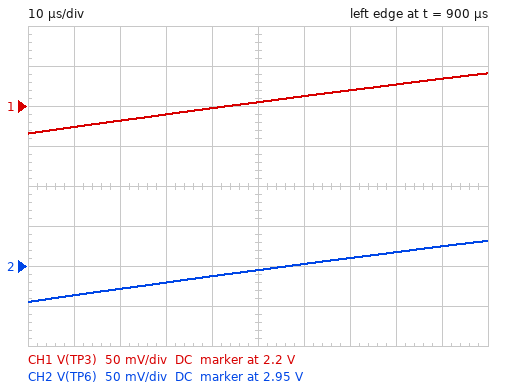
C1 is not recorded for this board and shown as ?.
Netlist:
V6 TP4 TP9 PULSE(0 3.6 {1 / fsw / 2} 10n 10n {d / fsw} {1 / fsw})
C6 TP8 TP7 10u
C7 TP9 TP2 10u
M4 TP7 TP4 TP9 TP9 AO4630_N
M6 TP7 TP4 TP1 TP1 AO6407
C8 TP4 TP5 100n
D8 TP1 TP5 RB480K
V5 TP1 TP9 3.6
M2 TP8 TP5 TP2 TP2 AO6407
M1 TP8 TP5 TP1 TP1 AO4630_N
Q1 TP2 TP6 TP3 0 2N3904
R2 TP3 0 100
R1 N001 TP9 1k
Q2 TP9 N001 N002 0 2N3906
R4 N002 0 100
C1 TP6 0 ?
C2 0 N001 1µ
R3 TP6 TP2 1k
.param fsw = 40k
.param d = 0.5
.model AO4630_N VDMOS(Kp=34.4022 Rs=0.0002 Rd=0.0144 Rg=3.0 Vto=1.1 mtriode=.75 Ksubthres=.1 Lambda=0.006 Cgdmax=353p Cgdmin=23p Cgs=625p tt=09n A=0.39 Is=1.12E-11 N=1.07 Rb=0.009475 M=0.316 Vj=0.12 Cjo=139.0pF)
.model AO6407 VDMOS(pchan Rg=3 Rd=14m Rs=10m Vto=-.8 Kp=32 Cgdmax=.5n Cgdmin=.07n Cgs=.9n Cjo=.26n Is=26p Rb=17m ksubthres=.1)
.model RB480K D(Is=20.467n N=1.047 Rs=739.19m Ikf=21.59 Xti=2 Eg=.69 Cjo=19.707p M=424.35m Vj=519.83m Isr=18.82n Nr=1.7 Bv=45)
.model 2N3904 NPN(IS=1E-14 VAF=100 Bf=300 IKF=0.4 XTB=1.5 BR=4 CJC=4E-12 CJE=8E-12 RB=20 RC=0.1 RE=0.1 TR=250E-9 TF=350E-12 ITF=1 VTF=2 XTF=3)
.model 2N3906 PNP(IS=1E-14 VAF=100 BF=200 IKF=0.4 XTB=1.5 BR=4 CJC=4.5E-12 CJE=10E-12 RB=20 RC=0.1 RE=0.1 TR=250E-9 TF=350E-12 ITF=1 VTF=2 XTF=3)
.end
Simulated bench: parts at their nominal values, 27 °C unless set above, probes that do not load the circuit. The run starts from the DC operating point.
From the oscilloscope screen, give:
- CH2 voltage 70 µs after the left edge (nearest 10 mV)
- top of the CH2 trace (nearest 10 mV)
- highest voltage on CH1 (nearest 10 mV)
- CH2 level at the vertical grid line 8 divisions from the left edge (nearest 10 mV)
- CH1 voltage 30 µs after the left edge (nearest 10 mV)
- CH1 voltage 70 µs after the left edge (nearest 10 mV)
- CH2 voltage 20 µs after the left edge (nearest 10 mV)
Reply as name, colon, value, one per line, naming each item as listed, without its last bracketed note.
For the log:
CH2 voltage 70 µs after the left edge: 2.96 V
top of the CH2 trace: 2.98 V
highest voltage on CH1: 2.24 V
CH2 level at the vertical grid line 8 divisions from the left edge: 2.97 V
CH1 voltage 30 µs after the left edge: 2.19 V
CH1 voltage 70 µs after the left edge: 2.22 V
CH2 voltage 20 µs after the left edge: 2.92 V
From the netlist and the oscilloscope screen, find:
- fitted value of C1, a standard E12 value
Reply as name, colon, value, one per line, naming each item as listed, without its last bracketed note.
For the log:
fitted value of C1, a standard E12 value: 330 nF
